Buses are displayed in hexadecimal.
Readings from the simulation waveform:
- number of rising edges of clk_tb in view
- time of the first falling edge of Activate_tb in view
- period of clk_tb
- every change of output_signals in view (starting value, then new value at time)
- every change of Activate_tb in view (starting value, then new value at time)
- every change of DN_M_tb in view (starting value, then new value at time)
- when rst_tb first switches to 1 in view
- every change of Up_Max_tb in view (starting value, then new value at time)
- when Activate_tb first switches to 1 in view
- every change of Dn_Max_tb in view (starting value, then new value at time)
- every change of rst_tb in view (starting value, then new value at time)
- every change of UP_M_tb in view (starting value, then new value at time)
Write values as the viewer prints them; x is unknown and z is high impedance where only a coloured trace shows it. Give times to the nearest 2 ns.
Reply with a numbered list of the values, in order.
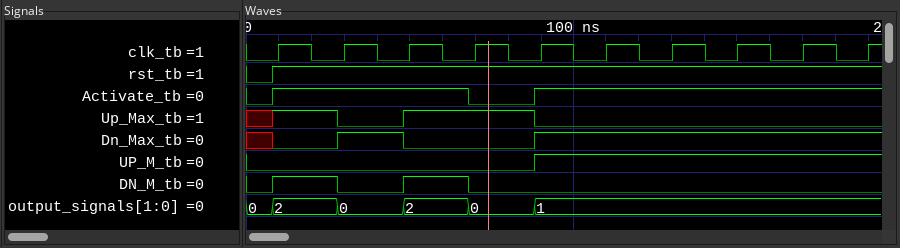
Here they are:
1. 10
2. 68 ns
3. 20 ns
4. 0, 2 at 8 ns, 0 at 28 ns, 2 at 48 ns, 0 at 68 ns, 1 at 88 ns
5. 0, 1 at 8 ns, 0 at 68 ns, 1 at 88 ns
6. 0, 1 at 8 ns, 0 at 28 ns, 1 at 48 ns, 0 at 68 ns
7. 8 ns
8. x, 1 at 8 ns, 0 at 28 ns, 1 at 48 ns, 0 at 88 ns
9. 8 ns
10. x, 0 at 8 ns, 1 at 28 ns, 0 at 48 ns, 1 at 88 ns
11. 0, 1 at 8 ns
12. 0, 1 at 88 ns
